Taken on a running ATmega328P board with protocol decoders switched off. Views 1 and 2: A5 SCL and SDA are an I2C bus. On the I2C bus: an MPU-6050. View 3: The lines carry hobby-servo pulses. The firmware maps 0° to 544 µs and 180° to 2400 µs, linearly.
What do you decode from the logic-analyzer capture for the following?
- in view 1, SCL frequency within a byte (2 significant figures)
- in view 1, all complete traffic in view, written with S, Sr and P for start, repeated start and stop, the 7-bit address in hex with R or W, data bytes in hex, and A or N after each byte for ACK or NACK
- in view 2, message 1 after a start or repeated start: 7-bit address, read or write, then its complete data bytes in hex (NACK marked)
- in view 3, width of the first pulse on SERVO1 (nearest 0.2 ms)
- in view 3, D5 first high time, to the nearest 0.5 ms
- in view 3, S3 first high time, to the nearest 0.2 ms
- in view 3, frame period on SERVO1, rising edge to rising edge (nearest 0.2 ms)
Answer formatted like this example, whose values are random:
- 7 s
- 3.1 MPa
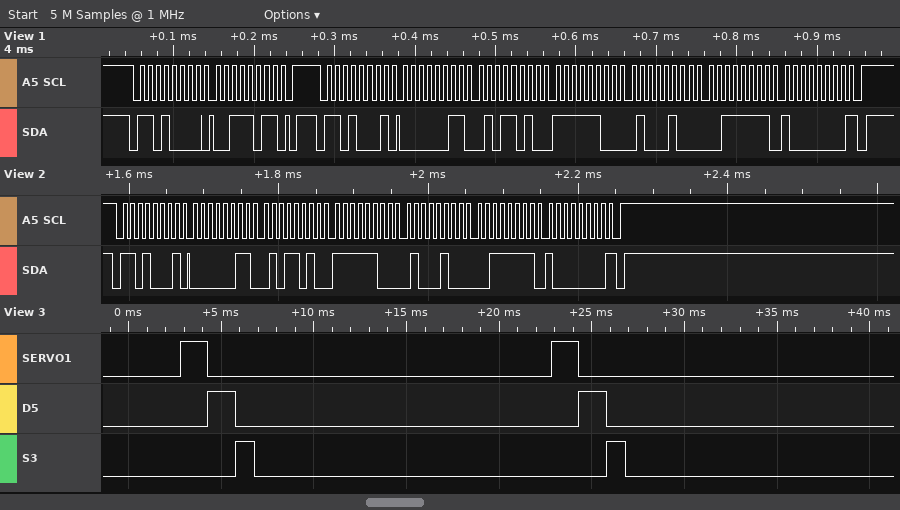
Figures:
- 100 kHz
- S 68W A 3B A P S 68R A 03 A 5A A FC A 44 A 3F A 80 N P
- 0x68 read: 03 5A FC 44 3F 80 NACK
- 1.4 ms
- 1.5 ms
- 1.0 ms
- 20.0 ms
